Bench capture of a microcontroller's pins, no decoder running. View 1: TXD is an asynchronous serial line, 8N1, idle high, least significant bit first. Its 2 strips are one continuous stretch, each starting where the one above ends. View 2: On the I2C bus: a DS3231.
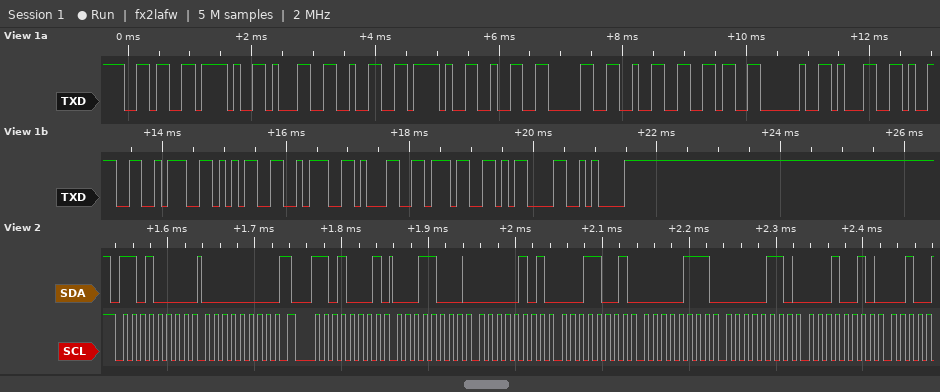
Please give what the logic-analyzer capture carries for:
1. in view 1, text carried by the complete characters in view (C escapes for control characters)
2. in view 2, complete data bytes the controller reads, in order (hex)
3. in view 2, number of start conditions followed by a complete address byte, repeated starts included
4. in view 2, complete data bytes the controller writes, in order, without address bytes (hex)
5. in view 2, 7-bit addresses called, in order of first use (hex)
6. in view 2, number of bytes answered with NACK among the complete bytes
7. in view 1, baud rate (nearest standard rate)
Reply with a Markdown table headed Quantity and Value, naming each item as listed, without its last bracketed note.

| Quantity | Value |
|---|---|
| in view 1, text carried by the complete characters in view | "6/12/2026 19:5:17\r\n" |
| in view 2, complete data bytes the controller reads, in order | 18 05 19 07 06 12 |
| in view 2, number of start conditions followed by a complete address byte, repeated starts included | 2 |
| in view 2, complete data bytes the controller writes, in order, without address bytes | 00 |
| in view 2, 7-bit addresses called, in order of first use | 0x68 |
| in view 2, number of bytes answered with NACK among the complete bytes | 0 |
| in view 1, baud rate | 9600 baud |
